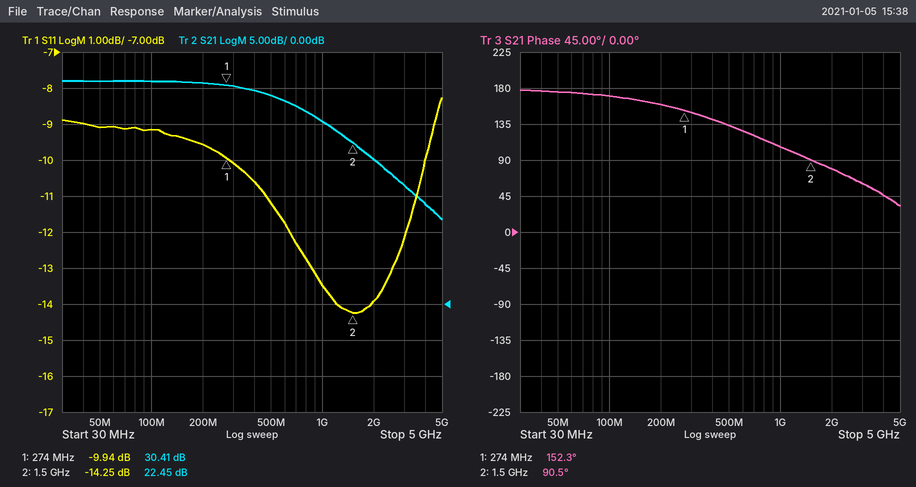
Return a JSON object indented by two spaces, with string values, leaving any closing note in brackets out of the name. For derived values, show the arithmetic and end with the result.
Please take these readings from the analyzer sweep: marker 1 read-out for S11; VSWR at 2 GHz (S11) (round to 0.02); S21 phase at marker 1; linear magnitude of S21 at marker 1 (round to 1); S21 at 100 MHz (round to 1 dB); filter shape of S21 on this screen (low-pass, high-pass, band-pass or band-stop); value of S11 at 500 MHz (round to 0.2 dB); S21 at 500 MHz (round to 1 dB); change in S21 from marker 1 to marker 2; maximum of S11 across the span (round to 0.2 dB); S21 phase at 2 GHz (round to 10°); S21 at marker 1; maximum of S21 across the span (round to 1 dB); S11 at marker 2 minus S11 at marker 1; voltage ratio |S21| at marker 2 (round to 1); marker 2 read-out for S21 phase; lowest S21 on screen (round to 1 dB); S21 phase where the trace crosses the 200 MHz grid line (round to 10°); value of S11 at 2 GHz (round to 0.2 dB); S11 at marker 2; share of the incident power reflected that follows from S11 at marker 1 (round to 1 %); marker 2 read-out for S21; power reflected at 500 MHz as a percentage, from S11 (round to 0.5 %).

{
  "marker 1 read-out for S11": "-9.94 dB",
  "VSWR at 2 GHz (S11)": "|Γ| = 10^(-14/20) = 0.1995; VSWR = (1 + 0.1995)/(1 − 0.1995) ≈ 1.50",
  "S21 phase at marker 1": "152.3°",
  "linear magnitude of S21 at marker 1": "10^(30.41/20) ≈ 33",
  "S21 at 100 MHz": "31 dB",
  "filter shape of S21 on this screen": "low-pass",
  "value of S11 at 500 MHz": "-11.2 dB",
  "S21 at 500 MHz": "29 dB",
  "change in S21 from marker 1 to marker 2": "22.45 − (30.41) = -7.96 dB",
  "maximum of S11 across the span": "-8.2 dB",
  "S21 phase at 2 GHz": "80°",
  "S21 at marker 1": "30.41 dB",
  "maximum of S21 across the span": "31 dB",
  "S11 at marker 2 minus S11 at marker 1": "-14.25 − (-9.94) = -4.31 dB",
  "voltage ratio |S21| at marker 2": "10^(22.45/20) ≈ 13",
  "marker 2 read-out for S21 phase": "90.5°",
  "lowest S21 on screen": "12 dB",
  "S21 phase where the trace crosses the 200 MHz grid line": "160°",
  "value of S11 at 2 GHz": "-14.0 dB",
  "S11 at marker 2": "-14.25 dB",
  "share of the incident power reflected that follows from S11 at marker 1": "10^(-9.94/10) ≈ 10 %",
  "marker 2 read-out for S21": "22.45 dB",
  "power reflected at 500 MHz as a percentage, from S11": "10^(-11.2/10) ≈ 7.59 %, so 7.5 % to the nearest 0.5 %"
}
